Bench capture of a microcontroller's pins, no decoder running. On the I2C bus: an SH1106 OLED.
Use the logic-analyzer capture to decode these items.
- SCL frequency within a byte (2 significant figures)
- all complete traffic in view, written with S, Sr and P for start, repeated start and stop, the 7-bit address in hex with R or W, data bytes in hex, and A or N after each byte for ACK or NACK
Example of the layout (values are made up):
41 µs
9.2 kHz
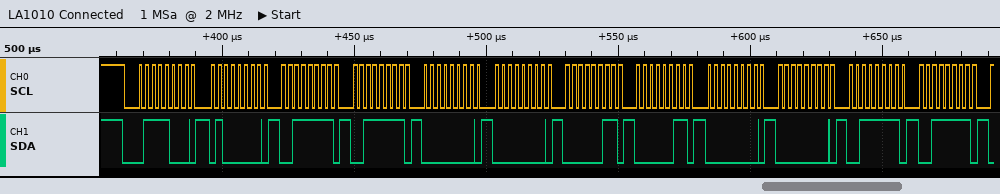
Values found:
400 kHz
S 3CW A 40 A 3F A 3F A 00 A 00 A 03 A 03 A 00 A 00 A 3F A 3F A
